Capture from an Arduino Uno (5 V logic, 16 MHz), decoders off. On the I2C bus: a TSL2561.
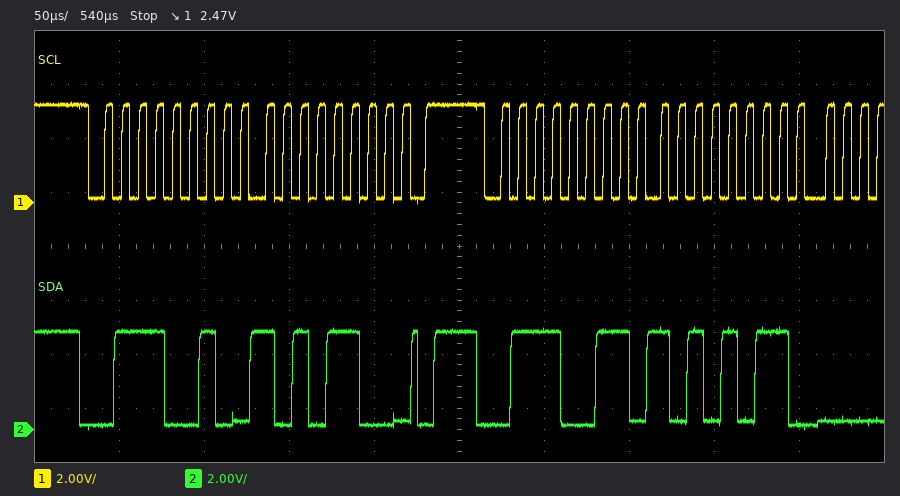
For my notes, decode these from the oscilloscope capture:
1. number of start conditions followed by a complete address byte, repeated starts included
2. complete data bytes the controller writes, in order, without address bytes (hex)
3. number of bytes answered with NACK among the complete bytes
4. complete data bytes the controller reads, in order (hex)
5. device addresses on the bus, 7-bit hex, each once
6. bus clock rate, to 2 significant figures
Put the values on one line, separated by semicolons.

2; AC; 0; AB; 0x39; 100 kHz
